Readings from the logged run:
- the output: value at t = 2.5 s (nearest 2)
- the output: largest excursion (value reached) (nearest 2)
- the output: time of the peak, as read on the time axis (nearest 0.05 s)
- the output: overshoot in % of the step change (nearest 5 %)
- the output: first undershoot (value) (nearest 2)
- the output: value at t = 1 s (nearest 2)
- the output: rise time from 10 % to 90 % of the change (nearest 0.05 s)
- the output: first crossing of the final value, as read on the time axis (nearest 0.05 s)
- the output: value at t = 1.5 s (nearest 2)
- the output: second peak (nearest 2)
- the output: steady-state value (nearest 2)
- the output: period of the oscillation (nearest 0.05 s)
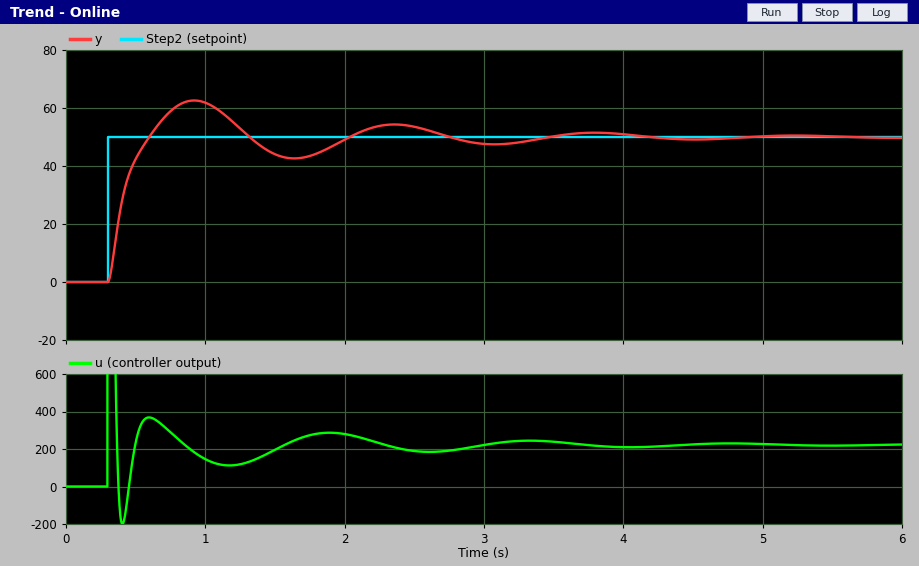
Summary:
54
62
0.90 s
25 %
42
62
0.20 s
0.60 s
44
54
50
1.45 s
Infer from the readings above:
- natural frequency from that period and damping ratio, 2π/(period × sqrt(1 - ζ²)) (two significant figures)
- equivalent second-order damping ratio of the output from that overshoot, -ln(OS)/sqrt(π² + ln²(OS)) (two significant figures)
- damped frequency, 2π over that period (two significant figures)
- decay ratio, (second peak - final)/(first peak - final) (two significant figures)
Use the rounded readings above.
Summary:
4.7 rad/s
0.40
4.3 rad/s
0.33
